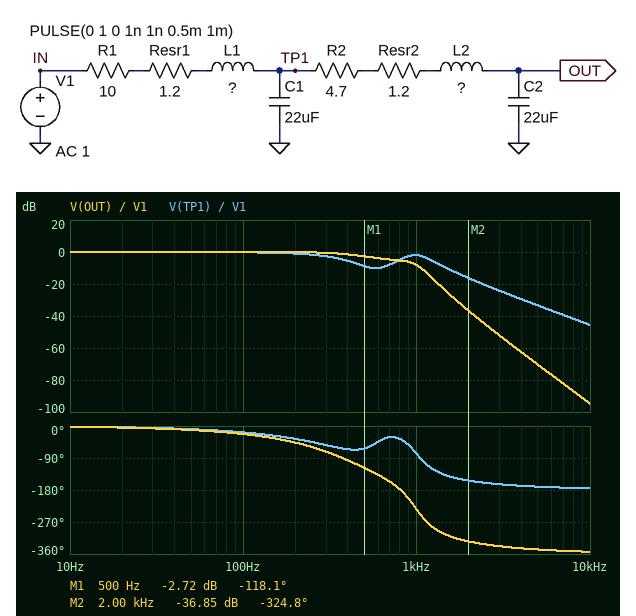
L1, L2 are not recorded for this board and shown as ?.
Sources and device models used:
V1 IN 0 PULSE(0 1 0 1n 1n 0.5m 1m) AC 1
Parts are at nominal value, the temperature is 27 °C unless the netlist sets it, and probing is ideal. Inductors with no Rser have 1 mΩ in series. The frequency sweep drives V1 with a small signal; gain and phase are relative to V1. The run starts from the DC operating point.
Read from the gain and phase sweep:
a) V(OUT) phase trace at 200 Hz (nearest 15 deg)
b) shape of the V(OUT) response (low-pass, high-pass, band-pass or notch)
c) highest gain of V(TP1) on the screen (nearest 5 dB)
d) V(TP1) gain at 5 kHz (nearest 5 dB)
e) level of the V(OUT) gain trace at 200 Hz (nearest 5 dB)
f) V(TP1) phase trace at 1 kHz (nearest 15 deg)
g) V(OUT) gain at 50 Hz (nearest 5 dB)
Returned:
-45 deg
low-pass
0 dB
-35 dB
0 dB
-75 deg
0 dB
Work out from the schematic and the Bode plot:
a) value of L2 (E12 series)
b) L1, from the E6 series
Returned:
3.3 mH
2.2 mH
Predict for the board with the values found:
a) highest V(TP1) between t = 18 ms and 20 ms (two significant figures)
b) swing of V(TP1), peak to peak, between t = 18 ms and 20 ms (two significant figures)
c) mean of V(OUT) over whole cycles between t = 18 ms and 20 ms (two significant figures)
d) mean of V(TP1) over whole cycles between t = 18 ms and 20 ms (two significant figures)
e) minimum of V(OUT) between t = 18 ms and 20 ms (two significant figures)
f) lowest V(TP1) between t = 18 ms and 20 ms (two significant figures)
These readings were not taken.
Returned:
1.0 V
1.0 V
500 mV
500 mV
250 mV
-2.7 mV
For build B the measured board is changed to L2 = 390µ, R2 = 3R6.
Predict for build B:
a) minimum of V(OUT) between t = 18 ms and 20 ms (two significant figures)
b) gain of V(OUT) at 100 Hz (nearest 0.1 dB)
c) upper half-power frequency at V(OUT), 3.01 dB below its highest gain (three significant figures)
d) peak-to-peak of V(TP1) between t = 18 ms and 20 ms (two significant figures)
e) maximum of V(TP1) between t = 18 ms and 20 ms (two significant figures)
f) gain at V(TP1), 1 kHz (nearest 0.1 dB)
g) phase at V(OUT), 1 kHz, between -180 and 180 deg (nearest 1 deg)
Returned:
340 mV
-0.2 dB
405 Hz
330 mV
670 mV
-12.7 dB
-151 deg
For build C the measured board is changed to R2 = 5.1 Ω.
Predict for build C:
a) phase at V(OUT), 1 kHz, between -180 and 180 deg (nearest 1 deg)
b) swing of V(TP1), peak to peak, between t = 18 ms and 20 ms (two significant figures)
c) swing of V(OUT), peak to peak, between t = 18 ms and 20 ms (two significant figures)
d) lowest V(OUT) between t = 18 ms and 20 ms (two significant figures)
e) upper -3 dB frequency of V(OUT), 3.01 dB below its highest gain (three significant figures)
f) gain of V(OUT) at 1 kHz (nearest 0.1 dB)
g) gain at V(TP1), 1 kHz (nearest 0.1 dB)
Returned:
126 deg
980 mV
480 mV
260 mV
511 Hz
-8.4 dB
-2.2 dB
